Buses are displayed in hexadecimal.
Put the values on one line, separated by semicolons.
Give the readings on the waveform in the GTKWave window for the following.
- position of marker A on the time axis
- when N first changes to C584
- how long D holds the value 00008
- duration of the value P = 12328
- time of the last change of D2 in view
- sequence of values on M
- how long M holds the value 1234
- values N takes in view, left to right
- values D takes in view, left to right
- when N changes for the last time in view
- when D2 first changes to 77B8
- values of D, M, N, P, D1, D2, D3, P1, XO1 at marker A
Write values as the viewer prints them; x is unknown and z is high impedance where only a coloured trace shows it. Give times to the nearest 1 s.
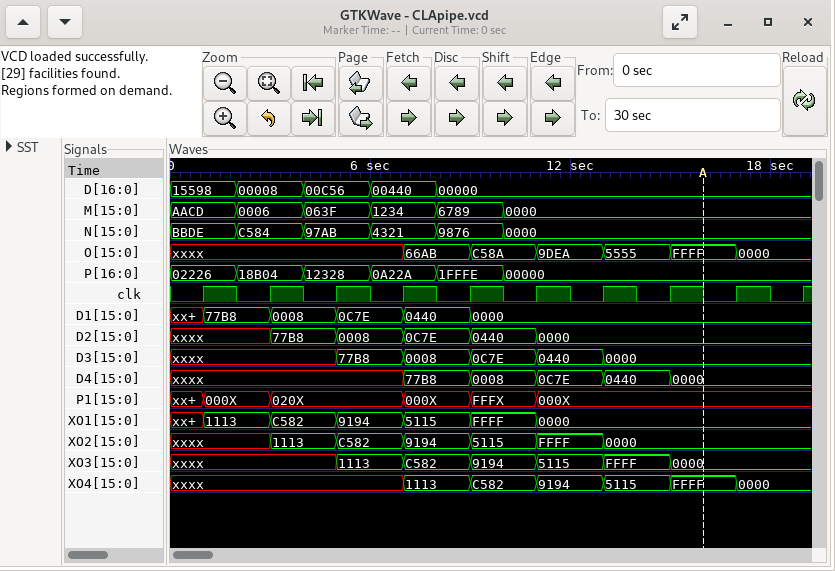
16 s; 2 s; 2 s; 2 s; 11 s; AACD, 0006, 063F, 1234, 6789, 0000; 2 s; BBDE, C584, 97AB, 4321, 9876, 0000; 15598, 00008, 00C56, 00440, 00000; 10 s; 3 s; D=00000, M=0000, N=0000, P=00000, D1=0000, D2=0000, D3=0000, P1=000X, XO1=0000
